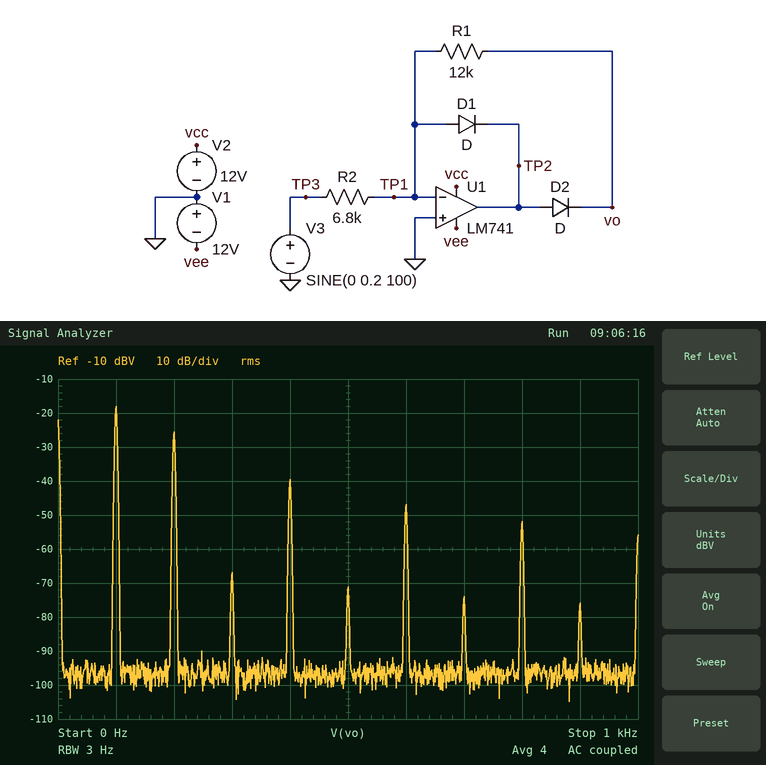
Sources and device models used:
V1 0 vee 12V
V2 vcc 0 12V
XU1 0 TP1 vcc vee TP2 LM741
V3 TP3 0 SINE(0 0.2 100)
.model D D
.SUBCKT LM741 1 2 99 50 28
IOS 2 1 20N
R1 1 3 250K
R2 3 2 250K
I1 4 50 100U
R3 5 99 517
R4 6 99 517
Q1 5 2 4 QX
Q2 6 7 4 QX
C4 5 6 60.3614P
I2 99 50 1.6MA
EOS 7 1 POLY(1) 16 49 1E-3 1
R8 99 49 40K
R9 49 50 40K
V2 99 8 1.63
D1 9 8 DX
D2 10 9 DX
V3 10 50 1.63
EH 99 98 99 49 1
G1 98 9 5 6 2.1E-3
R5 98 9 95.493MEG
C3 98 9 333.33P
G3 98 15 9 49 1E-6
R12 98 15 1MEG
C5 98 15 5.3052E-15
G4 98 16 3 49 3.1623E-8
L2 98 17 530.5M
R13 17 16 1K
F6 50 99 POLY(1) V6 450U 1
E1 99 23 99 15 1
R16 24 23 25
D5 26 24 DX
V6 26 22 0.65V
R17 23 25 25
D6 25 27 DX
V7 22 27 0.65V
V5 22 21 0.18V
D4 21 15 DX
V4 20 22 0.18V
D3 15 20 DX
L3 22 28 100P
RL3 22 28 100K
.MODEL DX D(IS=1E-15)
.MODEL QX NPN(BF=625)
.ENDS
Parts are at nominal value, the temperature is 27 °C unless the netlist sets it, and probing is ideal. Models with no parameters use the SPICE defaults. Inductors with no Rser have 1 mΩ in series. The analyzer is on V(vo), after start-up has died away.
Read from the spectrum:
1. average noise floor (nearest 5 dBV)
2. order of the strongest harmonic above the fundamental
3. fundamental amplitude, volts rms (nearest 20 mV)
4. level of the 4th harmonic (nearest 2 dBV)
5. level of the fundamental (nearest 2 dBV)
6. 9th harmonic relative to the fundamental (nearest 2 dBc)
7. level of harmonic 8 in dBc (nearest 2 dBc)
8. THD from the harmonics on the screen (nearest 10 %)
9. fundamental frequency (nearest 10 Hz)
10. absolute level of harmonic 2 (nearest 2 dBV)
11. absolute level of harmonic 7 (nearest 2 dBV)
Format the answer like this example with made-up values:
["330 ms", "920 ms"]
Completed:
["-95 dBV", "2", "120 mV", "-40 dBV", "-18 dBV", "-58 dBc", "-34 dBc", "40 %", "100 Hz", "-26 dBV", "-74 dBV"]
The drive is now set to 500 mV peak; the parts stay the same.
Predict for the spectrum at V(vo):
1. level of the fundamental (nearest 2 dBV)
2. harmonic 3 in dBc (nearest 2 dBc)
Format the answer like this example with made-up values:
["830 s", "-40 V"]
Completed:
["-10 dBV", "-56 dBc"]
